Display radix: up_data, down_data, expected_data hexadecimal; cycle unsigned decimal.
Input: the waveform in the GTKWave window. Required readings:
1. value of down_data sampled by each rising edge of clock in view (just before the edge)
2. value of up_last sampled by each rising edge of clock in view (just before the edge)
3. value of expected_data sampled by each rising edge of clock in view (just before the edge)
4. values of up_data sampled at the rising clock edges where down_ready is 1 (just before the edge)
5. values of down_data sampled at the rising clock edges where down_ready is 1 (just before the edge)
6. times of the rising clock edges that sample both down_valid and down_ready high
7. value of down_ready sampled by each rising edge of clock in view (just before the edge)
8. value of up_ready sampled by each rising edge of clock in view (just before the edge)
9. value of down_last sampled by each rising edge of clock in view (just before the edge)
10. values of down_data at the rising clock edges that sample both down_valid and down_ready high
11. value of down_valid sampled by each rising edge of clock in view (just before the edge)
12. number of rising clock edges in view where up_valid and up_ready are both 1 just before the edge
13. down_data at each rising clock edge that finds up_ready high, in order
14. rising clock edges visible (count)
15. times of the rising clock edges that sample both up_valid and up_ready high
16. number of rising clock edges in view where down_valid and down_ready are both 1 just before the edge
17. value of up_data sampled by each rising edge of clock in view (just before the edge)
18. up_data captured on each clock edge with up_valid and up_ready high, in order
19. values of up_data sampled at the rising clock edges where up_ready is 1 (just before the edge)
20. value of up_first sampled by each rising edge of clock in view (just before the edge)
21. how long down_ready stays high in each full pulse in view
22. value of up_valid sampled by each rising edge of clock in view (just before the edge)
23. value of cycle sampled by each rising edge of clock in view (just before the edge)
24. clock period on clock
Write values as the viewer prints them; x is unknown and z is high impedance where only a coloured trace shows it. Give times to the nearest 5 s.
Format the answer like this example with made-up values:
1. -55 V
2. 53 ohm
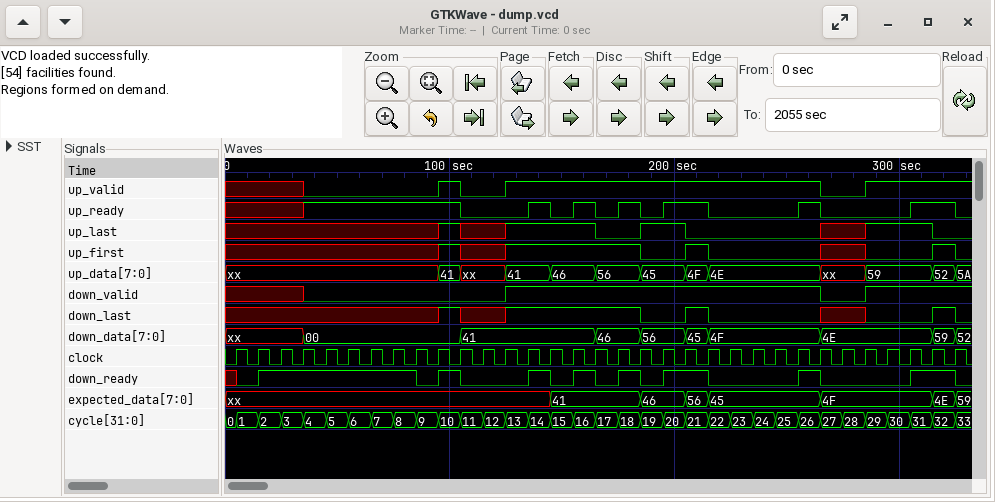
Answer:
1. xx, xx, xx, xx, 00, 00, 00, 00, 00, 00, 00, 41, 41, 41, 41, 41, 41, 46, 46, 56, 56, 45, 4F, 4F, 4F, 4F, 4F, 4E, 4E, 4E, 4E, 4E, 59
2. x x x x x x x x x x 1 x x 1 1 1 1 0 0 1 1 0 0 0 0 0 0 x x 1 1 1 0
3. xx, xx, xx, xx, xx, xx, xx, xx, xx, xx, xx, xx, xx, xx, xx, 41, 41, 41, 41, 46, 46, 56, 45, 45, 45, 45, 45, 4F, 4F, 4F, 4F, 4F, 4E
4. xx, xx, xx, xx, xx, xx, xx, 41, 41, 46, 56, 45, 4F, 4E, 59, 52
5. xx, xx, 00, 00, 00, 00, 00, 00, 41, 41, 46, 56, 45, 4F, 4E, 59
6. 145 s, 165 s, 185 s, 205 s, 215 s, 265 s, 315 s, 325 s
7. x 0 1 1 1 1 1 1 1 0 1 0 0 0 1 0 1 0 1 0 1 1 0 0 0 0 1 0 0 0 0 1 1
8. x x x x 1 1 1 1 1 1 1 0 0 0 1 0 1 0 1 0 1 1 0 0 0 0 1 0 0 0 0 1 1
9. x x x x x x x x x x 1 x x 1 1 1 1 1 1 0 0 1 0 0 0 0 0 x x 0 0 0 1
10. 41, 41, 46, 56, 45, 4F, 4E, 59
11. x x x x 0 0 0 0 0 0 0 0 0 1 1 1 1 1 1 1 1 1 1 1 1 1 1 0 0 1 1 1 1
12. 9
13. 00, 00, 00, 00, 00, 00, 00, 41, 41, 46, 56, 45, 4F, 4E, 59
14. 33
15. 105 s, 145 s, 165 s, 185 s, 205 s, 215 s, 265 s, 315 s, 325 s
16. 8
17. xx, xx, xx, xx, xx, xx, xx, xx, xx, xx, 41, xx, xx, 41, 41, 46, 46, 56, 56, 45, 45, 4F, 4E, 4E, 4E, 4E, 4E, xx, xx, 59, 59, 59, 52
18. 41, 41, 46, 56, 45, 4F, 4E, 59, 52
19. xx, xx, xx, xx, xx, xx, 41, 41, 46, 56, 45, 4F, 4E, 59, 52
20. x x x x x x x x x x 1 x x 1 1 1 1 1 1 0 0 1 0 0 0 0 0 x x 0 0 0 1
21. 70 s, 10 s, 10 s, 10 s, 10 s, 20 s, 10 s, 20 s
22. x x x x 0 0 0 0 0 0 1 0 0 1 1 1 1 1 1 1 1 1 1 1 1 1 1 0 0 1 1 1 1
23. 0, 1, 2, 3, 4, 5, 6, 7, 8, 9, 10, 11, 12, 13, 14, 15, 16, 17, 18, 19, 20, 21, 22, 23, 24, 25, 26, 27, 28, 29, 30, 31, 32
24. 10 s
